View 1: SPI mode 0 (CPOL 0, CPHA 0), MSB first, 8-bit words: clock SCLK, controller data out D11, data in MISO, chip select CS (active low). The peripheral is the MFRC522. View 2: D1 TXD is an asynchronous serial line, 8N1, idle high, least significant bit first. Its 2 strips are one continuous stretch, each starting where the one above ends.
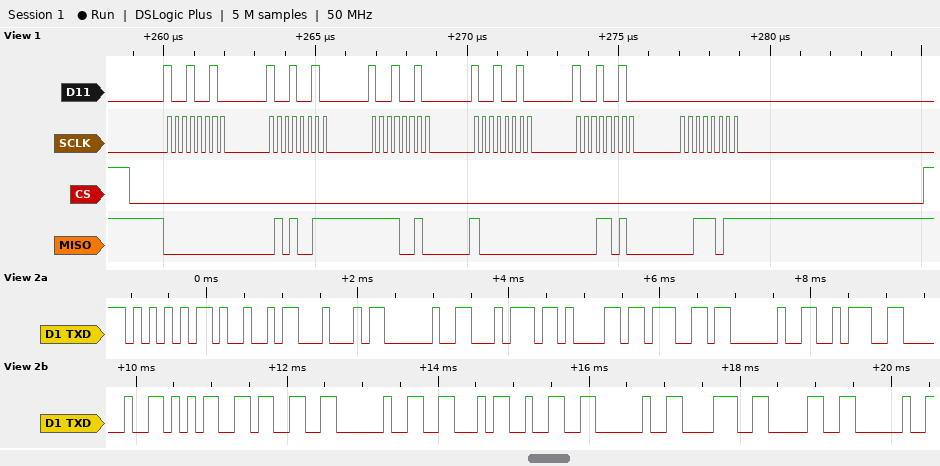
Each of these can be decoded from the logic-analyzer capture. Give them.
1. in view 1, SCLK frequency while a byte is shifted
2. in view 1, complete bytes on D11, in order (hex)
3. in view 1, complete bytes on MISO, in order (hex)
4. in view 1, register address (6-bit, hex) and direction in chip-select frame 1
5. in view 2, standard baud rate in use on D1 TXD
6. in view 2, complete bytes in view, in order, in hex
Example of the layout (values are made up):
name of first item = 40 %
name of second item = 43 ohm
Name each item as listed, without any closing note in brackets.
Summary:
in view 1, SCLK frequency while a byte is shifted = 4 MHz
in view 1, complete bytes on D11, in order = 0x92 0x92 0x92 0x92 0x92 0x00
in view 1, complete bytes on MISO, in order = 0x00 0x53 0xF2 0x80 0x1A 0x3B
in view 1, register address (6-bit, hex) and direction in chip-select frame 1 = 0x09 read
in view 2, standard baud rate in use on D1 TXD = 9600 baud
in view 2, complete bytes in view, in order, in hex = 0x55 0x49 0x44 0x20 0x74 0x61 0x67 0x20 0x3A 0x20 0x35 0x33 0x20 0x46 0x32 0x20 0x38 0x30 0x20
